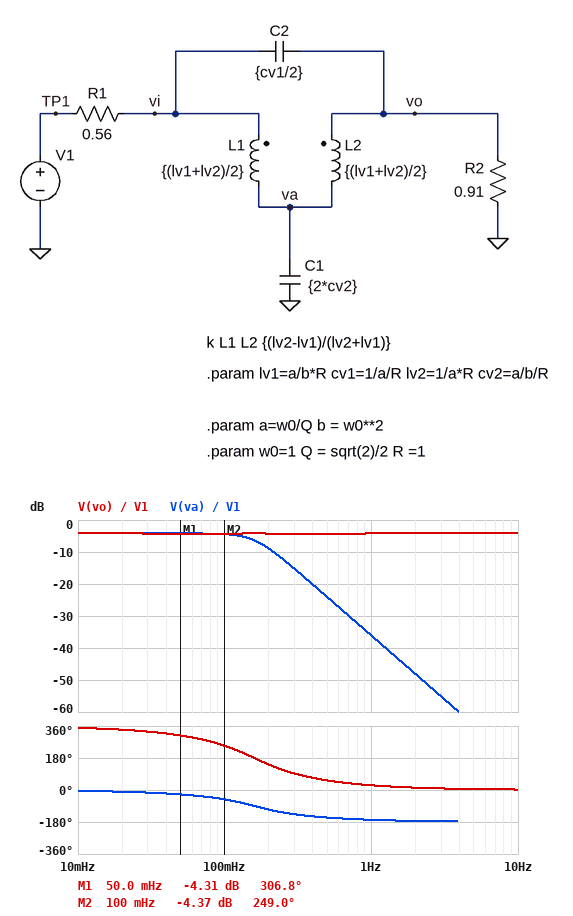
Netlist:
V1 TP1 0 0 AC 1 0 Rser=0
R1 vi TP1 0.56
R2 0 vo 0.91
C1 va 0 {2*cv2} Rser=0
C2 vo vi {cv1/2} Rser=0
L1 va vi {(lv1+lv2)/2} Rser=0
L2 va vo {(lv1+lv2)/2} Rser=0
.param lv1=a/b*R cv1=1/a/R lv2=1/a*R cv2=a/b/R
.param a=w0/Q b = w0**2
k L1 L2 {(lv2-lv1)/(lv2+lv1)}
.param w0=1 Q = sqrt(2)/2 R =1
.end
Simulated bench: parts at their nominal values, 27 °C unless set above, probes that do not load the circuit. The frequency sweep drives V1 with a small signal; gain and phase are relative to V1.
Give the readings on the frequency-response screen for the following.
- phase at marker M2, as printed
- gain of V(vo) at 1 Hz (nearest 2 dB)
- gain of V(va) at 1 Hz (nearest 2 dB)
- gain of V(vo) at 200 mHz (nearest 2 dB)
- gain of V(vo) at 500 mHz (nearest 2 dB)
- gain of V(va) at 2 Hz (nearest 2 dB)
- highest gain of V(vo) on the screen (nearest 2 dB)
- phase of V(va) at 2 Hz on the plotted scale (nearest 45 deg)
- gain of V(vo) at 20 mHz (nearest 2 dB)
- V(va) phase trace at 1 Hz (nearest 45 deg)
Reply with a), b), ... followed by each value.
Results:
a) 249.0 deg
b) -4 dB
c) -36 dB
d) -4 dB
e) -4 dB
f) -48 dB
g) -4 dB
h) -180 deg
i) -4 dB
j) -180 deg
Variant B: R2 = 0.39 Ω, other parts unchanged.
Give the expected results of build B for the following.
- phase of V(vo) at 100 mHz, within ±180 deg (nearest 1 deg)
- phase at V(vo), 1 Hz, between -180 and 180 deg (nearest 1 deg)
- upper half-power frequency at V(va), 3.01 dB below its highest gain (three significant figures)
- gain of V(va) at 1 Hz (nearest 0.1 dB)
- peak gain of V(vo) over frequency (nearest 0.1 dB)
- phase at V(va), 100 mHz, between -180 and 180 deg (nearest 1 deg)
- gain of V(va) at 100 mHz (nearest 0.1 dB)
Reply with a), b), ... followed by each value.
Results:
a) -107 deg
b) 32 deg
c) 189 mHz
d) -39.1 dB
e) -7.7 dB
f) -32 deg
g) -3.5 dB
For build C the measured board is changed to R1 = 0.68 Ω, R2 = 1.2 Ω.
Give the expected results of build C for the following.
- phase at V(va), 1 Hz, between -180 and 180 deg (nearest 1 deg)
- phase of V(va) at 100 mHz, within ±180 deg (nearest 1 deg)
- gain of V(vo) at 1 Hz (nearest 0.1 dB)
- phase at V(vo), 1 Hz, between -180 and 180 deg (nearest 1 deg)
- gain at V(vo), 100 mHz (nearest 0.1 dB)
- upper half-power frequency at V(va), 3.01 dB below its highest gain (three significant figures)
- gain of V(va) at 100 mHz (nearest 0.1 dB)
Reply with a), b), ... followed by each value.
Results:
a) -166 deg
b) -61 deg
c) -3.8 dB
d) 25 deg
e) -3.6 dB
f) 131 mHz
g) -5.3 dB
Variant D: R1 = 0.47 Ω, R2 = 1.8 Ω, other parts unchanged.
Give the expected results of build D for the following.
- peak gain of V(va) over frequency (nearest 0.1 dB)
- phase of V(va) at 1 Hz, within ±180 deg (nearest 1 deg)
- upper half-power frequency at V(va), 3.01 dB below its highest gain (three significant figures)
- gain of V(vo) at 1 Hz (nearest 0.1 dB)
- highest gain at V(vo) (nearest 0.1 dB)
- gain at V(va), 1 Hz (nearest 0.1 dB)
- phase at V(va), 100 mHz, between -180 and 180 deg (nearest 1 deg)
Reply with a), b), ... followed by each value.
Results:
a) -1.6 dB
b) -166 deg
c) 106 mHz
d) -1.7 dB
e) -0.2 dB
f) -33.8 dB
g) -77 deg
